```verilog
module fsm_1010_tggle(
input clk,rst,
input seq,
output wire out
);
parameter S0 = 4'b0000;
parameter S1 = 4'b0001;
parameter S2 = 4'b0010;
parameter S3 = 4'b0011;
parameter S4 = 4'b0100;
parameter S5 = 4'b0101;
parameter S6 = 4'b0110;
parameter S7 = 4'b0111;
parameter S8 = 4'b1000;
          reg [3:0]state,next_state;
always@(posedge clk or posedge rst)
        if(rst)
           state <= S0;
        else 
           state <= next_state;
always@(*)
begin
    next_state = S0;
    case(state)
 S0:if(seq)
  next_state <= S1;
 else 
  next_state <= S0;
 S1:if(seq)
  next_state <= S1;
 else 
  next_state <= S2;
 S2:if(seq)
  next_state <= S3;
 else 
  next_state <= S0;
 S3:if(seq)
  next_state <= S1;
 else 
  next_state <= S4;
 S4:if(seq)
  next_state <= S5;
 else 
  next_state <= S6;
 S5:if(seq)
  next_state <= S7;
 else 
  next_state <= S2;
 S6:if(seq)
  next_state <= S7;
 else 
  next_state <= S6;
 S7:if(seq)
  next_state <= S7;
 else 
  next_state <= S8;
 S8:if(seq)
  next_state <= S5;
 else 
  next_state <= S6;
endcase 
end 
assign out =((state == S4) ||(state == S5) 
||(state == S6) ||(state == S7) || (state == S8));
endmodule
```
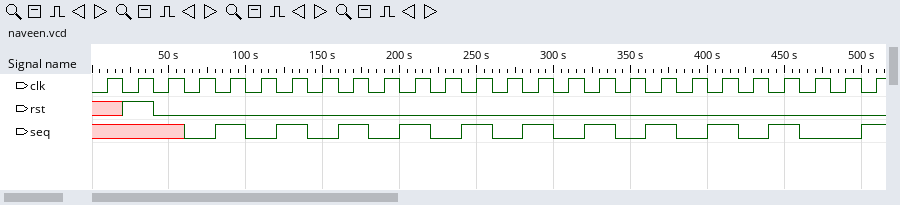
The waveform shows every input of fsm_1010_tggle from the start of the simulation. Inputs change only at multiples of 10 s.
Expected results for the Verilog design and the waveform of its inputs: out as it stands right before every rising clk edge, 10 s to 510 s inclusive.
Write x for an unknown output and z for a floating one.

x 0 0 0 0 0 0 0 1 1 0 0 1 1 0 0 1 1 0 0 1 1 0 0 1 1
